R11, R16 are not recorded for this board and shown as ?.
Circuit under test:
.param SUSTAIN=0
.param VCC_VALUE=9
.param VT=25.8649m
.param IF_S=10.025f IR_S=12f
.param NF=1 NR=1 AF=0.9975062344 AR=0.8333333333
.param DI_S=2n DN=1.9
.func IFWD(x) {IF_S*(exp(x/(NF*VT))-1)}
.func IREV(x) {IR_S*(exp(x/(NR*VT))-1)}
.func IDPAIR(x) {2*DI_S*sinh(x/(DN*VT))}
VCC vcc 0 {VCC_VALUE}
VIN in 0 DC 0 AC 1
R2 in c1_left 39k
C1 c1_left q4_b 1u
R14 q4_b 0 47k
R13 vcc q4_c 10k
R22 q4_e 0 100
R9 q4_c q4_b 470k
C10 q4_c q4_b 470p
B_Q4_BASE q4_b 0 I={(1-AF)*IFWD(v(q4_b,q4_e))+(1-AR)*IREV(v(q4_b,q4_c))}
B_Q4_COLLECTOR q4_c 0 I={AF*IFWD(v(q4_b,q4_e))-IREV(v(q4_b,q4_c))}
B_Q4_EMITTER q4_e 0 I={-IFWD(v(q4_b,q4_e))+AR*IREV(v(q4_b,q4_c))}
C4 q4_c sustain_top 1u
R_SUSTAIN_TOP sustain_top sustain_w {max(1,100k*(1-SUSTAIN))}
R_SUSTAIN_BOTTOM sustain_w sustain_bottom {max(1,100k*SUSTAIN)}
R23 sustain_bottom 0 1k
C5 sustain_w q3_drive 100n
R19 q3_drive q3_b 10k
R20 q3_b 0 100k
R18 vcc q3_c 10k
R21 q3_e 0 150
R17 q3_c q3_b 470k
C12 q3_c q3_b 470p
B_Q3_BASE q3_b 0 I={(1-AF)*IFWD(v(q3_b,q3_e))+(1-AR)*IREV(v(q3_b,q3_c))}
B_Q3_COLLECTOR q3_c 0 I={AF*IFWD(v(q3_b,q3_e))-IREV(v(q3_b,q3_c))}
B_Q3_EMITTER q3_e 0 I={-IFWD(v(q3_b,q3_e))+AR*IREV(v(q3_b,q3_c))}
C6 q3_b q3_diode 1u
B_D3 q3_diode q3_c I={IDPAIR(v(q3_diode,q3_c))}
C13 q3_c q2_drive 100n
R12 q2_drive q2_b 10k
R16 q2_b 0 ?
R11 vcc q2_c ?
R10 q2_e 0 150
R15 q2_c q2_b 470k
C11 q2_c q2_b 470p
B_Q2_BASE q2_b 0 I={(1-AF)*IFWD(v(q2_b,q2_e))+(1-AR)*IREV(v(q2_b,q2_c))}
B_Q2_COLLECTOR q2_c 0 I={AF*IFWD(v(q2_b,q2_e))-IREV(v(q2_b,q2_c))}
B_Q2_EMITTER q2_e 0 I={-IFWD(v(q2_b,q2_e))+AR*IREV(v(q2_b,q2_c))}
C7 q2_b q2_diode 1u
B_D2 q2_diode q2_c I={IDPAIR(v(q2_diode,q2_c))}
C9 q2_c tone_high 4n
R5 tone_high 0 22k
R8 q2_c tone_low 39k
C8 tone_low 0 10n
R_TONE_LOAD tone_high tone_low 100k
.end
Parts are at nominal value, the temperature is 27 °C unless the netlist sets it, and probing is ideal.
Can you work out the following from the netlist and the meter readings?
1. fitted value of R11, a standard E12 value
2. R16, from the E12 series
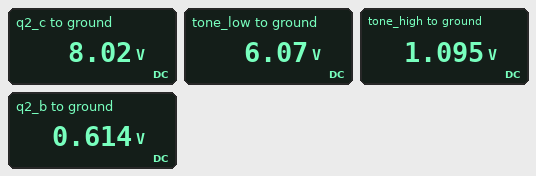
15 kΩ
39 kΩ
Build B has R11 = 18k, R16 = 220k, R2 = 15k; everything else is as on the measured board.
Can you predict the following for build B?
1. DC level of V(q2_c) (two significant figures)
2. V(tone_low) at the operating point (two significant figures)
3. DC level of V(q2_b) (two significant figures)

7.9 V
6.0 V
2.5 V
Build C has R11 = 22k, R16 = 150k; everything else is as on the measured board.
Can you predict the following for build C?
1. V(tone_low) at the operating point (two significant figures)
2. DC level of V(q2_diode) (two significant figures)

5.8 V
7.7 V
